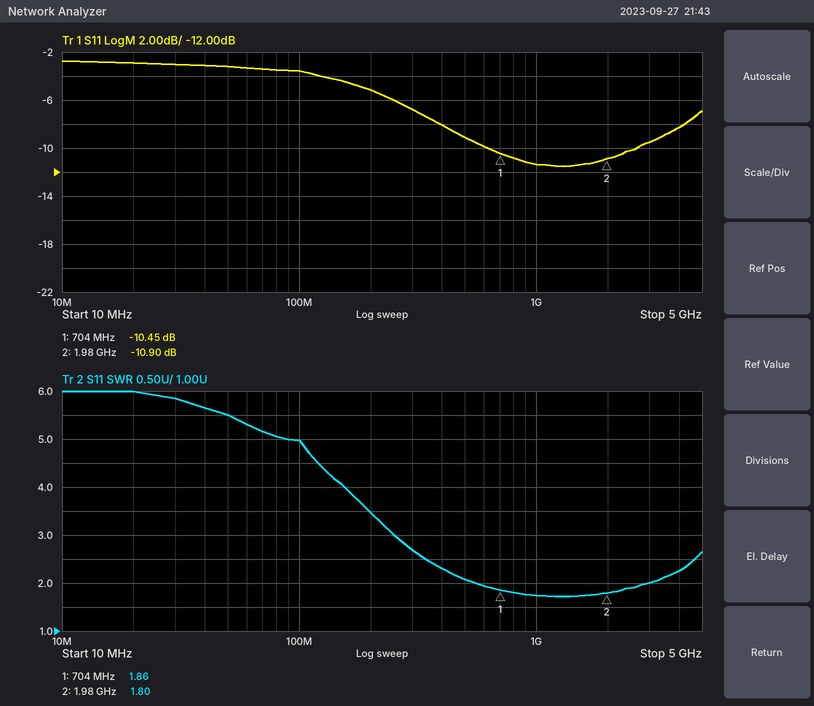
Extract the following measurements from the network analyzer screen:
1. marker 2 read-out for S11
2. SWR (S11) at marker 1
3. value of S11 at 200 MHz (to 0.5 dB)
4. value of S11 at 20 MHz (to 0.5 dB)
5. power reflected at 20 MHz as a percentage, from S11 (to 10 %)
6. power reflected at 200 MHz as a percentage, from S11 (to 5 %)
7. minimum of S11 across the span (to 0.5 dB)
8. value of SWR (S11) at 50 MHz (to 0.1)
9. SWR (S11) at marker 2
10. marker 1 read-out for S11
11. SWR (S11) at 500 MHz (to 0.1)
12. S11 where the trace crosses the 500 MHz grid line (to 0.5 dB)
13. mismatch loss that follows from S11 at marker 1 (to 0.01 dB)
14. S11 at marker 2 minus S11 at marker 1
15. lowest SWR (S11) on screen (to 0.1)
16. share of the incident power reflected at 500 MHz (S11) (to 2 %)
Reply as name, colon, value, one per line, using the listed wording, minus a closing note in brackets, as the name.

marker 2 read-out for S11: -10.90 dB
SWR (S11) at marker 1: 1.86
value of S11 at 200 MHz: -5.0 dB
value of S11 at 20 MHz: -3.0 dB
power reflected at 20 MHz as a percentage, from S11: 50 %
power reflected at 200 MHz as a percentage, from S11: 30 %
minimum of S11 across the span: -11.5 dB
value of SWR (S11) at 50 MHz: 5.5
SWR (S11) at marker 2: 1.80
marker 1 read-out for S11: -10.45 dB
SWR (S11) at 500 MHz: 2.1
S11 where the trace crosses the 500 MHz grid line: -9.0 dB
mismatch loss that follows from S11 at marker 1: 0.41 dB
S11 at marker 2 minus S11 at marker 1: -0.45 dB
lowest SWR (S11) on screen: 1.7
share of the incident power reflected at 500 MHz (S11): 12 %
